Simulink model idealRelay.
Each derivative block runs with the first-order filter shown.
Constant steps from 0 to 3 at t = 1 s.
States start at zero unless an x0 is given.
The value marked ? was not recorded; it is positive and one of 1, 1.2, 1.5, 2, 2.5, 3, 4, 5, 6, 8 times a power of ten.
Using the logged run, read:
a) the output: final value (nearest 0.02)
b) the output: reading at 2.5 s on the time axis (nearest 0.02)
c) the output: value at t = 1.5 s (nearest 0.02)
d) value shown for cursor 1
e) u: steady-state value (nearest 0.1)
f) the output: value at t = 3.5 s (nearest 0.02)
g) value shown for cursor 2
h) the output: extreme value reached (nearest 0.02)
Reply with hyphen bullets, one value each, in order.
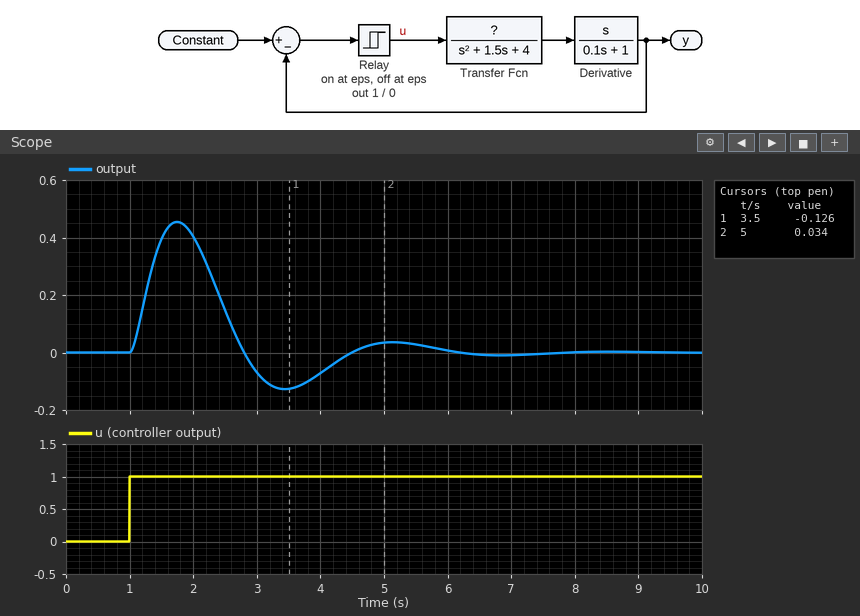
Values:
- 0.00
- 0.14
- 0.40
- -0.126
- 1.0
- -0.12
- 0.034
- 0.46
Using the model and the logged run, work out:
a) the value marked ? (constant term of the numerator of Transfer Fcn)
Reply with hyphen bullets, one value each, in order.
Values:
- 1.5
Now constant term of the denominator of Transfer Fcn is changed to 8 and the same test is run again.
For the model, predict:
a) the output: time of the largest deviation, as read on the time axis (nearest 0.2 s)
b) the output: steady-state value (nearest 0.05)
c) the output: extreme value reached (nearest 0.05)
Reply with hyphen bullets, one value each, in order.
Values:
- 1.6 s
- 0.00
- 0.35
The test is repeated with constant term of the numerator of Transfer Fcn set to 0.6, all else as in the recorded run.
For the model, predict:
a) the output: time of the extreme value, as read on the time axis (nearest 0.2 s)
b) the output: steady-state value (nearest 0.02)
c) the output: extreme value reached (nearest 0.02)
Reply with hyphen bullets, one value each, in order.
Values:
- 1.8 s
- 0.00
- 0.18
